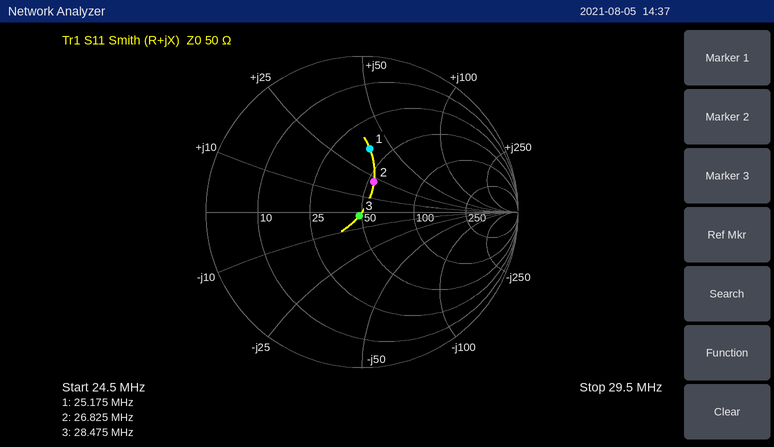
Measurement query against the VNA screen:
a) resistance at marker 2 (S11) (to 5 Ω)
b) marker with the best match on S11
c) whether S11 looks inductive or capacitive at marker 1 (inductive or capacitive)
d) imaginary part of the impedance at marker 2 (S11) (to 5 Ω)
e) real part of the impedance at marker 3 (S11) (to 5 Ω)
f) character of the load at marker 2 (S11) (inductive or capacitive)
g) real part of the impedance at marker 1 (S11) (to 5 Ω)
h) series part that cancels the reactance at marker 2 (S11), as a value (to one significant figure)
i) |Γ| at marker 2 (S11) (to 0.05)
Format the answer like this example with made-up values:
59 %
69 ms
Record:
55 Ω
marker 3
inductive
+20 Ω
50 Ω
inductive
40 Ω
300 pF
0.20
